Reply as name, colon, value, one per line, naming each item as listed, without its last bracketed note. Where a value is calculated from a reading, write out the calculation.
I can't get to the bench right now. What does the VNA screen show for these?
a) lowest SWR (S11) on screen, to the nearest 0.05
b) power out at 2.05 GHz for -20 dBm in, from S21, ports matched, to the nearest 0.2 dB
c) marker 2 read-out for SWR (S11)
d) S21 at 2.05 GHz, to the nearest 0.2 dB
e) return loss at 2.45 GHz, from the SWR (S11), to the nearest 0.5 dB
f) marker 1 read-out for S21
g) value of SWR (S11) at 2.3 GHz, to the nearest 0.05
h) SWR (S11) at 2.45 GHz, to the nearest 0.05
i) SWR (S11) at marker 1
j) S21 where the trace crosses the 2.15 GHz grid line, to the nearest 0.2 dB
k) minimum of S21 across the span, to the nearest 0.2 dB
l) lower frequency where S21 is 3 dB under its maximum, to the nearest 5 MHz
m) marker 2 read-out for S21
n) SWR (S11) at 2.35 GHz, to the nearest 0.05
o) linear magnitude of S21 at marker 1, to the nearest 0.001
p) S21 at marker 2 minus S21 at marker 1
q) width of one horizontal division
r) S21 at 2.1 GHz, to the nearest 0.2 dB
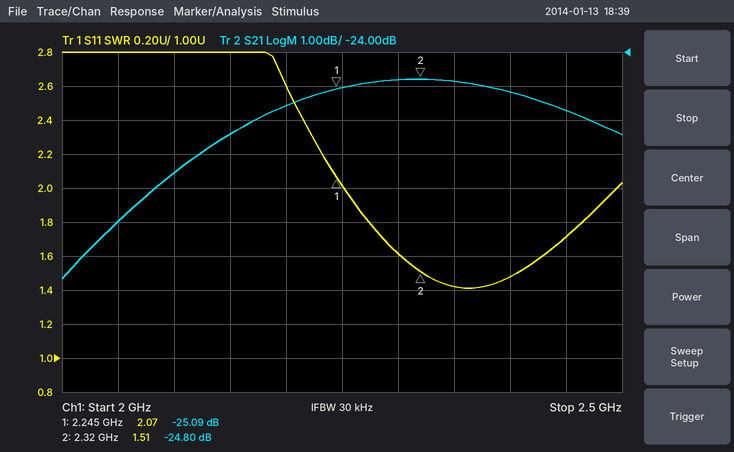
lowest SWR (S11) on screen, to the nearest 0.05: 1.40
power out at 2.05 GHz for -20 dBm in, from S21, ports matched, to the nearest 0.2 dB: -20 dBm + (-29.0 dB) = -49.0 dBm
marker 2 read-out for SWR: 1.51
S21 at 2.05 GHz, to the nearest 0.2 dB: -29.0 dB
return loss at 2.45 GHz, from the SWR (S11), to the nearest 0.5 dB: −20 log10((1.7 − 1)/(1.7 + 1)) ≈ 11.7 dB, so 11.5 dB to the nearest 0.5 dB
marker 1 read-out for S21: -25.09 dB
value of SWR (S11) at 2.3 GHz, to the nearest 0.05: 1.60
SWR (S11) at 2.45 GHz, to the nearest 0.05: 1.70
SWR (S11) at marker 1: 2.07
S21 where the trace crosses the 2.15 GHz grid line, to the nearest 0.2 dB: -26.4 dB
minimum of S21 across the span, to the nearest 0.2 dB: -30.6 dB
lower frequency where S21 is 3 dB under its maximum, to the nearest 5 MHz: 2.090 GHz
marker 2 read-out for S21: -24.80 dB
SWR (S11) at 2.35 GHz, to the nearest 0.05: 1.40
linear magnitude of S21 at marker 1, to the nearest 0.001: 10^(-25.09/20) ≈ 0.056
S21 at marker 2 minus S21 at marker 1: -24.8 − (-25.09) = 0.29 dB
width of one horizontal division: 50 MHz
S21 at 2.1 GHz, to the nearest 0.2 dB: -27.6 dB
